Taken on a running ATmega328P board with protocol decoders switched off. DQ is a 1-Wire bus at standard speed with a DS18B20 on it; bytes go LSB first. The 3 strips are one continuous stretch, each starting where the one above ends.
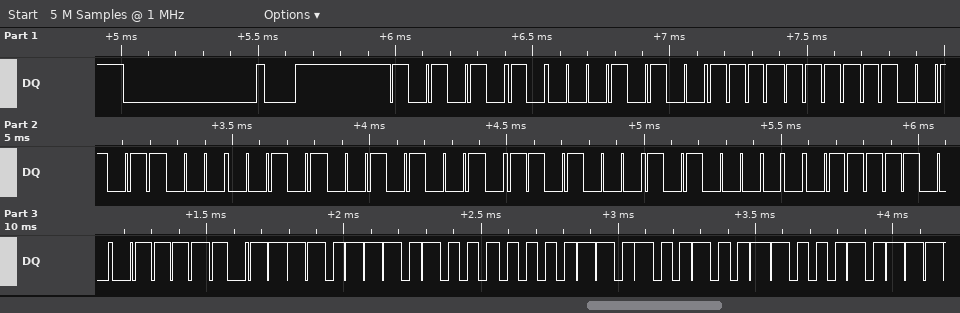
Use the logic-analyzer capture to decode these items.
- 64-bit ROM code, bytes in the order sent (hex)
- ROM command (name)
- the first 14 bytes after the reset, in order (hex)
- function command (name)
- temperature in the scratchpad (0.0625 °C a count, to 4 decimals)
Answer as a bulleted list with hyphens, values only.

- 28 FF D3 A0 94 16 05 3E
- Match ROM
- 55 28 FF D3 A0 94 16 05 3E BE 77 01 4B 46
- Read Scratchpad
- 23.4375 °C
